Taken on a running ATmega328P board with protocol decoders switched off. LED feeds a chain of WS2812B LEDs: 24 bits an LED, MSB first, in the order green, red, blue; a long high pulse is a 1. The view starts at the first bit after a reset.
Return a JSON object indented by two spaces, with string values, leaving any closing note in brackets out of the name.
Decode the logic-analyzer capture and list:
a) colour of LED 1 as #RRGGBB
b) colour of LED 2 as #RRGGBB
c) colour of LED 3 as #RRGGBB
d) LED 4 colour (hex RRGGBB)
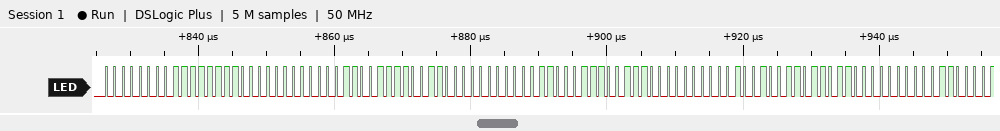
{
  "colour of LED 1 as #RRGGBB": "#FF0000",
  "colour of LED 2 as #RRGGBB": "#F30C00",
  "colour of LED 3 as #RRGGBB": "#E71800",
  "LED 4 colour": "#DB2400"
}
